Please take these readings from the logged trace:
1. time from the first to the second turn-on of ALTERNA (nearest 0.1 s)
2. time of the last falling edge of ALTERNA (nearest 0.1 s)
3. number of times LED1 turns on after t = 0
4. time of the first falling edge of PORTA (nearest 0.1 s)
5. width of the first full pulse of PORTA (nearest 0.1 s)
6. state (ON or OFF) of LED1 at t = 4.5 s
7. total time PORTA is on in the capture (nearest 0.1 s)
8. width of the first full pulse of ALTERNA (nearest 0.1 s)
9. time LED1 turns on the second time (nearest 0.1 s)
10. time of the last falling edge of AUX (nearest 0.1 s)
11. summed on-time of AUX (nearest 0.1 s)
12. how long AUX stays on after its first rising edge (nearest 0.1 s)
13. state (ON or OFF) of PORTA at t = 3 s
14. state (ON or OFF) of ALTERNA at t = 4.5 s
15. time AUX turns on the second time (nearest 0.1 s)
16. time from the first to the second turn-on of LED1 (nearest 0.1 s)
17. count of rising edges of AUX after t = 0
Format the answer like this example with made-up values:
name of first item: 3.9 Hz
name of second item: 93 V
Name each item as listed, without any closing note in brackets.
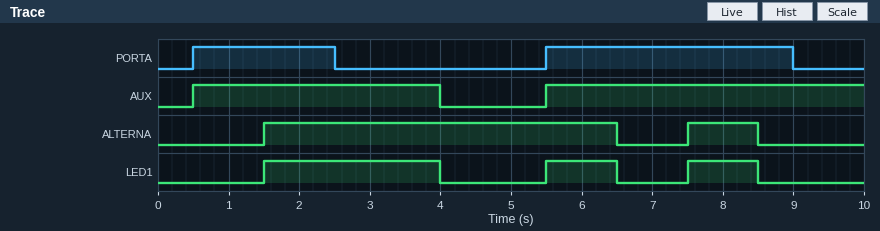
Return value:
time from the first to the second turn-on of ALTERNA: 6.0 s
time of the last falling edge of ALTERNA: 8.5 s
number of times LED1 turns on after t = 0: 3
time of the first falling edge of PORTA: 2.5 s
width of the first full pulse of PORTA: 2.0 s
state (ON or OFF) of LED1 at t = 4.5 s: OFF
total time PORTA is on in the capture: 5.5 s
width of the first full pulse of ALTERNA: 5.0 s
time LED1 turns on the second time: 5.5 s
time of the last falling edge of AUX: 4.0 s
summed on-time of AUX: 8.0 s
how long AUX stays on after its first rising edge: 3.5 s
state (ON or OFF) of PORTA at t = 3 s: OFF
state (ON or OFF) of ALTERNA at t = 4.5 s: ON
time AUX turns on the second time: 5.5 s
time from the first to the second turn-on of LED1: 4.0 s
count of rising edges of AUX after t = 0: 2
